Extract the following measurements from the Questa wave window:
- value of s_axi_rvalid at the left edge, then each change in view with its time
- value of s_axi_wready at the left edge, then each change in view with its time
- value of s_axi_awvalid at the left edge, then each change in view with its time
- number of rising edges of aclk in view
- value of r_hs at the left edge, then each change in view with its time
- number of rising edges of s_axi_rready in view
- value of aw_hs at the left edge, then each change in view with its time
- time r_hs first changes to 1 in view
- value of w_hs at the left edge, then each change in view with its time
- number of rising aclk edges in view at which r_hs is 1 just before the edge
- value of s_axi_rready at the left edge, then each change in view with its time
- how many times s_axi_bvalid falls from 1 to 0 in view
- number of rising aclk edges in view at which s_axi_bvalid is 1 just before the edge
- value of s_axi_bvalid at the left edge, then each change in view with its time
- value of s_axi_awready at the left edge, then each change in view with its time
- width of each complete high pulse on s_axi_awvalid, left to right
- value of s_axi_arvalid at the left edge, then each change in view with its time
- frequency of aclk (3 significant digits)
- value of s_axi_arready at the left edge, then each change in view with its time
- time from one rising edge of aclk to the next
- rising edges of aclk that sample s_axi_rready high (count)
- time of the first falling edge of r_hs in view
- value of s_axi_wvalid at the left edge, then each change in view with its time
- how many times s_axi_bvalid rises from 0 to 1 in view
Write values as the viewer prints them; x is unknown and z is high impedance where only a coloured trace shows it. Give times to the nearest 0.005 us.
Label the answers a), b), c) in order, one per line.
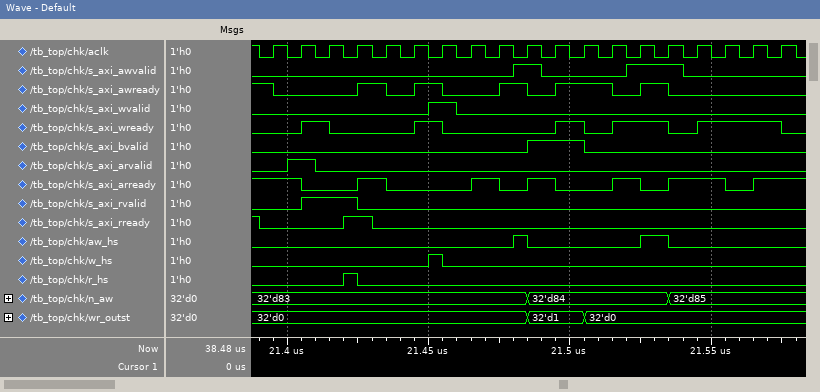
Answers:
a) 0, 1 at 21.405 us, 0 at 21.425 us
b) 0, 1 at 21.405 us, 0 at 21.415 us, 1 at 21.445 us, 0 at 21.455 us, 1 at 21.495 us, 0 at 21.505 us, 1 at 21.515 us, 0 at 21.535 us, 1 at 21.545 us, 0 at 21.575 us
c) 0, 1 at 21.48 us, 0 at 21.49 us, 1 at 21.52 us, 0 at 21.54 us
d) 19
e) 0, 1 at 21.42 us, 0 at 21.425 us
f) 1
g) 0, 1 at 21.48 us, 0 at 21.485 us, 1 at 21.525 us, 0 at 21.535 us
h) 21.42 us
i) 0, 1 at 21.45 us, 0 at 21.455 us
j) 1
k) 1, 0 at 21.39 us, 1 at 21.42 us, 0 at 21.43 us
l) 1
m) 2
n) 0, 1 at 21.485 us, 0 at 21.505 us
o) 1, 0 at 21.395 us, 1 at 21.425 us, 0 at 21.435 us, 1 at 21.445 us, 0 at 21.455 us, 1 at 21.475 us, 0 at 21.485 us, 1 at 21.495 us, 0 at 21.515 us, 1 at 21.525 us, 0 at 21.535 us
p) 0.01 us, 0.02 us
q) 0, 1 at 21.4 us, 0 at 21.41 us
r) 100 MHz
s) 1, 0 at 21.405 us, 1 at 21.425 us, 0 at 21.435 us, 1 at 21.465 us, 0 at 21.475 us, 1 at 21.485 us, 0 at 21.495 us, 1 at 21.515 us, 0 at 21.525 us, 1 at 21.535 us, 0 at 21.555 us, 1 at 21.565 us
t) 0.01 us
u) 1
v) 21.425 us
w) 0, 1 at 21.45 us, 0 at 21.46 us
x) 1
